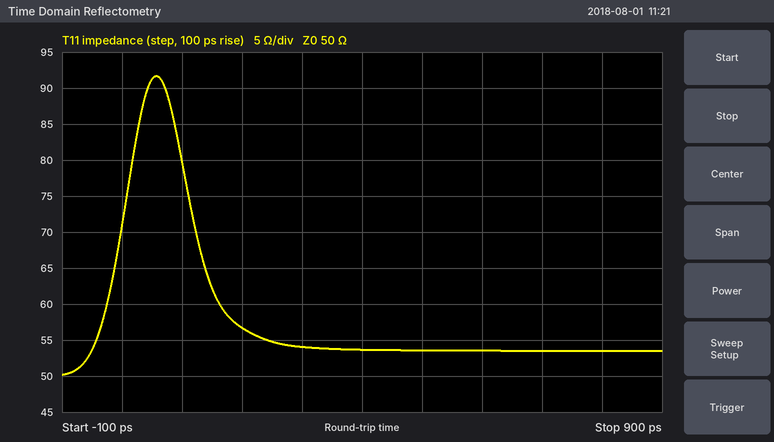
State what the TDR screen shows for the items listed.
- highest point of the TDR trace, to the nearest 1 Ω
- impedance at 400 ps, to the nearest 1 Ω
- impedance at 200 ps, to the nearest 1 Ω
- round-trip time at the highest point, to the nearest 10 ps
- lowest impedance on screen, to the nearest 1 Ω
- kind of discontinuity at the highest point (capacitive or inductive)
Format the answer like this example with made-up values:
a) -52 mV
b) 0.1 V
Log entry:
a) 92 Ω
b) 54 Ω
c) 57 Ω
d) 60 ps
e) 50 Ω
f) inductive
